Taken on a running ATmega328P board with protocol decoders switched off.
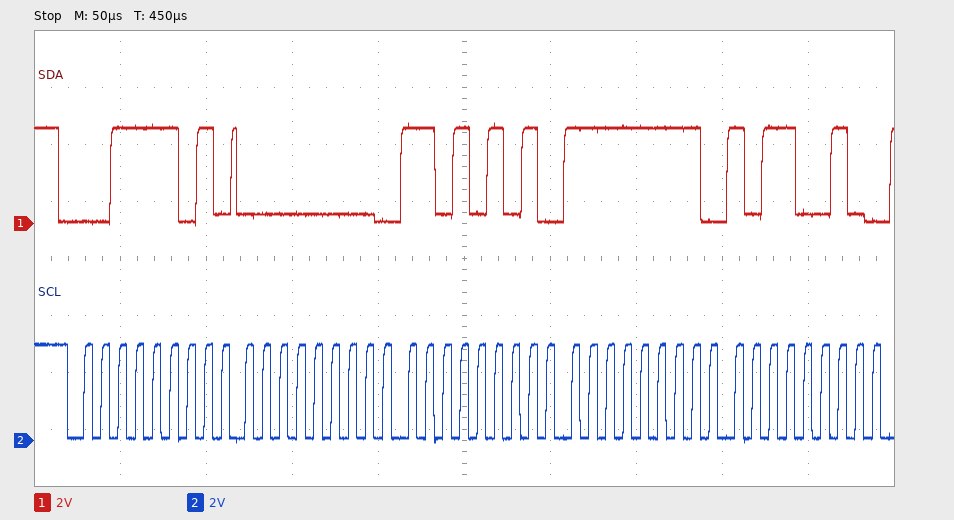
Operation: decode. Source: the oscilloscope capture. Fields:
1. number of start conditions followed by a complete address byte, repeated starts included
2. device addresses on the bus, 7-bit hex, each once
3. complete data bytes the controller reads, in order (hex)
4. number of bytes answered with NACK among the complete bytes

1
0x1E
00 D5 FF B2
0
